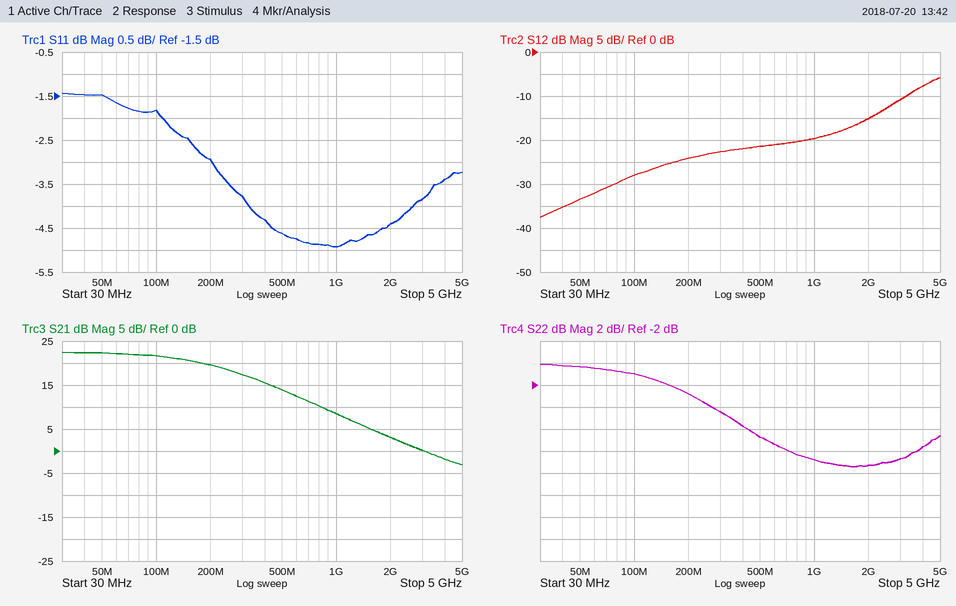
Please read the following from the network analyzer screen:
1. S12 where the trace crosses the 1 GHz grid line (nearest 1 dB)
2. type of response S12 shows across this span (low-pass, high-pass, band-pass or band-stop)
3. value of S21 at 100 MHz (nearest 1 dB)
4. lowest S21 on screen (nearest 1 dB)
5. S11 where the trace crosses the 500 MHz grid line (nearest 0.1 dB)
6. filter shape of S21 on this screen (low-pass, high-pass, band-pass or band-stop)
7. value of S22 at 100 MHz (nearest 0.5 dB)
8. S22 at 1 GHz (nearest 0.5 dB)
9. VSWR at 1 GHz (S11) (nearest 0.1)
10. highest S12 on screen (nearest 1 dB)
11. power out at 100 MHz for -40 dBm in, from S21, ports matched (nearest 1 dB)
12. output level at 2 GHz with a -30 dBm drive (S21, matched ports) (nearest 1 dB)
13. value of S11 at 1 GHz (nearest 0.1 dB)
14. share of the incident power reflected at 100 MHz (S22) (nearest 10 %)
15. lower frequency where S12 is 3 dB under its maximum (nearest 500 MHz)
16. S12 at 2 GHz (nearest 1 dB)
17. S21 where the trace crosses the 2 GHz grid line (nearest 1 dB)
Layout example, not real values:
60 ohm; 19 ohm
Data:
-20 dB; high-pass; 22 dB; -3 dB; -4.6 dB; low-pass; -1.0 dB; -9.0 dB; 3.6; -6 dB; -18 dBm; -27 dBm; -4.9 dB; 80 %; 3.5 GHz; -15 dB; 3 dB
